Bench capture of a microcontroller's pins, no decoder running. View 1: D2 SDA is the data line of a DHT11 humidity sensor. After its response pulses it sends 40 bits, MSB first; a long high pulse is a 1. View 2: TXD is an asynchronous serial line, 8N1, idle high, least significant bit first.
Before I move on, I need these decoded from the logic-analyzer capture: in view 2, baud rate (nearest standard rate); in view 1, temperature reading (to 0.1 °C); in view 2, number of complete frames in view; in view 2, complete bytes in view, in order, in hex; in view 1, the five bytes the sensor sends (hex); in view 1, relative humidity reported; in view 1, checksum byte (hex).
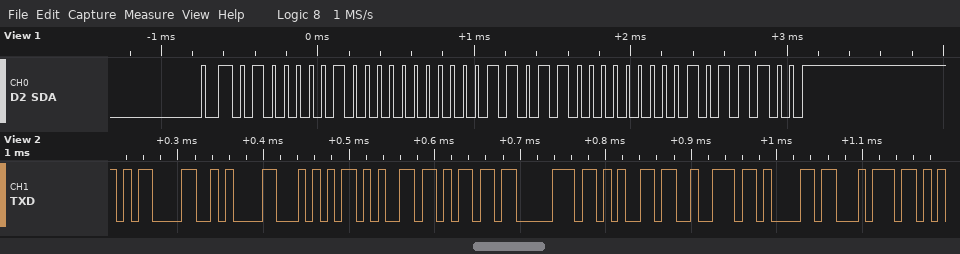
115200 baud
27.0 °C
10
0D 0A 54 65 6D 70 65 72 61 74
41 00 1B 00 5C
65 %
0x5C
